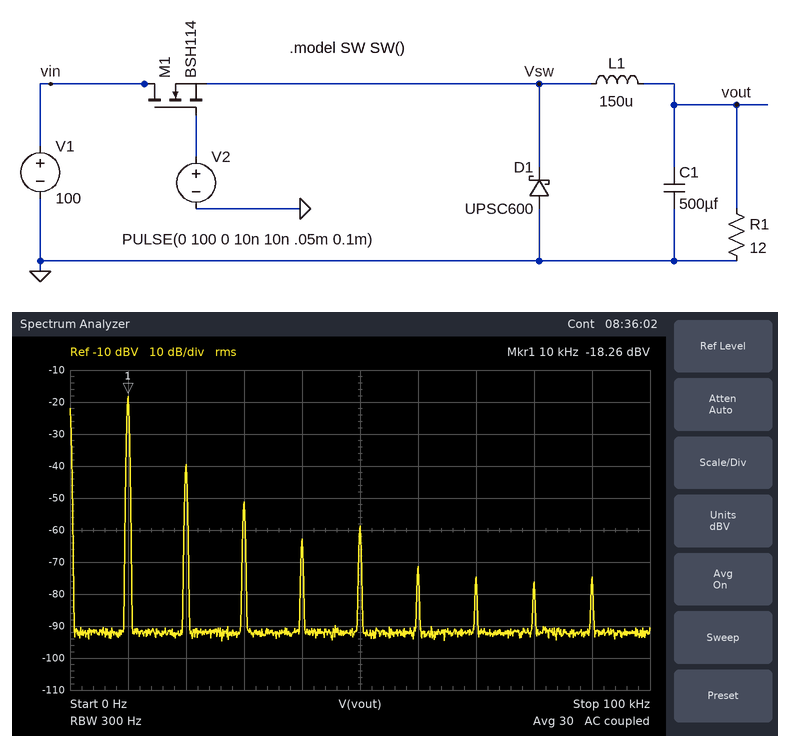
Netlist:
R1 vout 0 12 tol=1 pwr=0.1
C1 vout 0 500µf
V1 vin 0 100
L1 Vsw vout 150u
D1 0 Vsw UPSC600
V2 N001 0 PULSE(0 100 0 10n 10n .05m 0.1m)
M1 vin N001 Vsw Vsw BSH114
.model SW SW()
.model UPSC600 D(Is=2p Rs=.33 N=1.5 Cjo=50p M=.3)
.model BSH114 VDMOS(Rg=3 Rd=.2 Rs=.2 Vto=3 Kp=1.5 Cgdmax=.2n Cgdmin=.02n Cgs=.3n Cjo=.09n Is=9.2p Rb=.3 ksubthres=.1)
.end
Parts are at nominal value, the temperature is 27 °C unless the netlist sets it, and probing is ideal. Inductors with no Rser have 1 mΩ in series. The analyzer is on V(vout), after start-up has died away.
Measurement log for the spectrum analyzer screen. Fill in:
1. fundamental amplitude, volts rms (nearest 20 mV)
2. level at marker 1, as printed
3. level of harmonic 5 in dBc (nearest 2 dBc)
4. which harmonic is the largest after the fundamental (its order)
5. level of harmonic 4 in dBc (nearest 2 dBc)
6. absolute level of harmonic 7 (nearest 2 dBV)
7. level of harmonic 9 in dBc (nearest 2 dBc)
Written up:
120 mV
-18.26 dBV
-40 dBc
2
-44 dBc
-74 dBV
-56 dBc
